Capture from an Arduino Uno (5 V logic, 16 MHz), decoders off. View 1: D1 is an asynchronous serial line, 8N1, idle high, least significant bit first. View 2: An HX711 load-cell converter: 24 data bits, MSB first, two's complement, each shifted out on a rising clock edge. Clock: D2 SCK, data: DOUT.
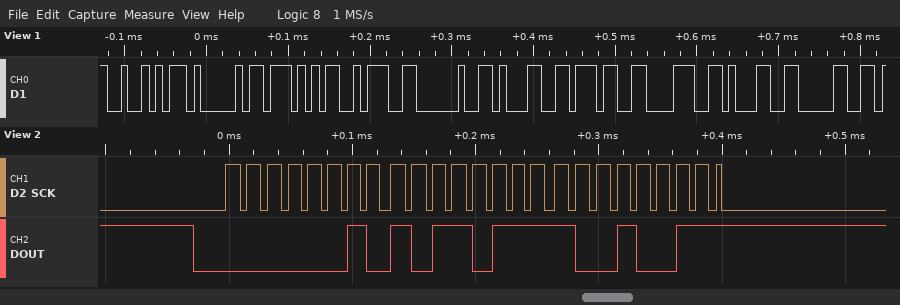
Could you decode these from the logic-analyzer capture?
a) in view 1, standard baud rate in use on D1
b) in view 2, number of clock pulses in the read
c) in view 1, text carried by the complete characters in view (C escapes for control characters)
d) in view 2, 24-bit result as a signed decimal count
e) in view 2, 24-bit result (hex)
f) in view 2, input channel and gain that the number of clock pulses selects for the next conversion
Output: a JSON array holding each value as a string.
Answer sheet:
["115200 baud", "25", "\"RAW: 17810\"", "178067", "0x02B793", "channel A, gain 128"]
